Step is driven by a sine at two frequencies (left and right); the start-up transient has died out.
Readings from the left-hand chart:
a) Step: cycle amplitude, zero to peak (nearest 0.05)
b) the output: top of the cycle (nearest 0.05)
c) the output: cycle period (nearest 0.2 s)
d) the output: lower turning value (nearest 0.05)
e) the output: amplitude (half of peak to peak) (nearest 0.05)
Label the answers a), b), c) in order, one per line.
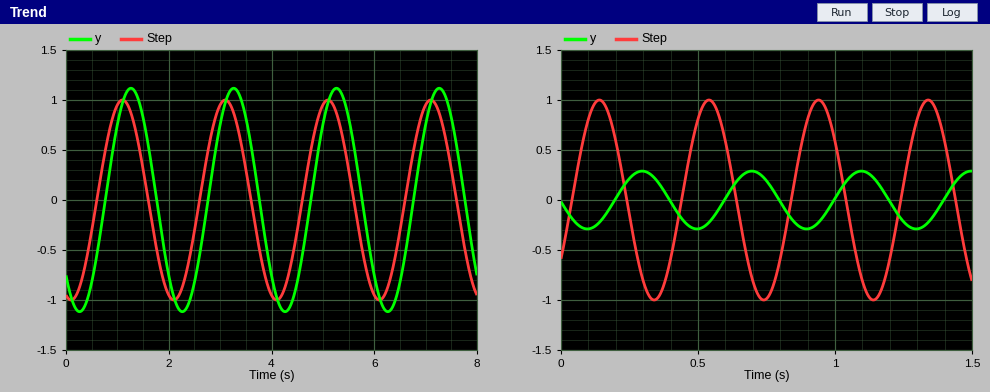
a) 1.00
b) 1.10
c) 2.0 s
d) -1.10
e) 1.10
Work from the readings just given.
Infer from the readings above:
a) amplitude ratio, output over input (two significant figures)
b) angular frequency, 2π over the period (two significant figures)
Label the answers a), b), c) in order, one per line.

a) 1.1
b) 3.1 rad/s
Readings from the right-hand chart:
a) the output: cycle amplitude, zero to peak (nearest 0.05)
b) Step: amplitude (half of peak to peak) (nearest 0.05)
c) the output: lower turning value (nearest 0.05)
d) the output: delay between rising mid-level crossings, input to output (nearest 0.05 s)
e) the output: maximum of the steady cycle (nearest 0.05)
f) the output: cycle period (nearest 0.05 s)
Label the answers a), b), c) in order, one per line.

a) 0.30
b) 1.00
c) -0.30
d) 0.15 s
e) 0.30
f) 0.40 s
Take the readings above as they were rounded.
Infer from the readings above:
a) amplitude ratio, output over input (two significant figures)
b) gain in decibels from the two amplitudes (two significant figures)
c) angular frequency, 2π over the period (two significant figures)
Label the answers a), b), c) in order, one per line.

a) 0.30
b) -10 dB
c) 16 rad/s
